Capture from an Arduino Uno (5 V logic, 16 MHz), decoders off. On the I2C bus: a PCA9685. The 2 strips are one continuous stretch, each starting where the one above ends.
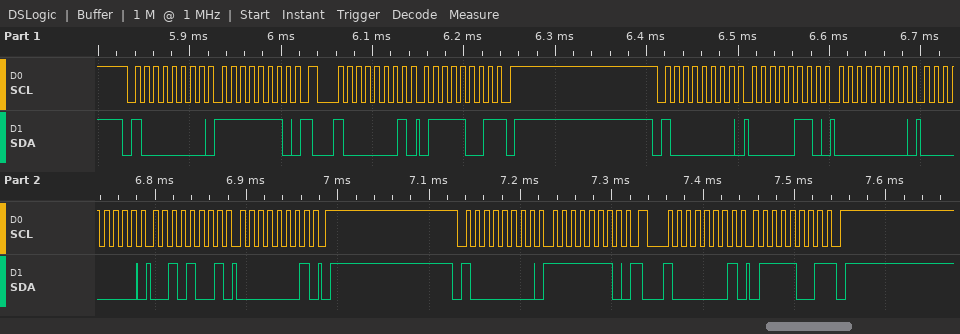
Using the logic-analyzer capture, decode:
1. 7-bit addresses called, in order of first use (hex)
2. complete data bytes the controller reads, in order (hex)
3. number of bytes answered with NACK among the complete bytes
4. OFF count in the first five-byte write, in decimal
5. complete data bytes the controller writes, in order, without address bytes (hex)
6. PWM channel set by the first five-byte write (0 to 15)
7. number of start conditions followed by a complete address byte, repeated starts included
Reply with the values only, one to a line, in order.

0x40
79 79
2
297
FE 06 00 00 29 01 FE
0
5
